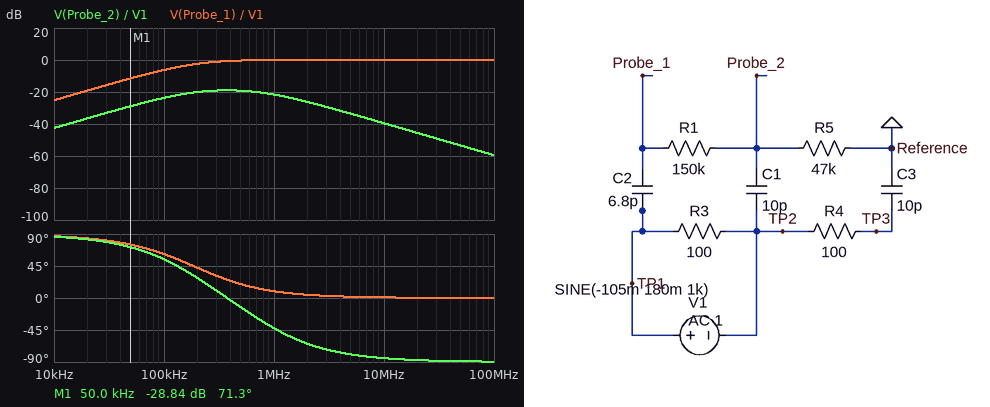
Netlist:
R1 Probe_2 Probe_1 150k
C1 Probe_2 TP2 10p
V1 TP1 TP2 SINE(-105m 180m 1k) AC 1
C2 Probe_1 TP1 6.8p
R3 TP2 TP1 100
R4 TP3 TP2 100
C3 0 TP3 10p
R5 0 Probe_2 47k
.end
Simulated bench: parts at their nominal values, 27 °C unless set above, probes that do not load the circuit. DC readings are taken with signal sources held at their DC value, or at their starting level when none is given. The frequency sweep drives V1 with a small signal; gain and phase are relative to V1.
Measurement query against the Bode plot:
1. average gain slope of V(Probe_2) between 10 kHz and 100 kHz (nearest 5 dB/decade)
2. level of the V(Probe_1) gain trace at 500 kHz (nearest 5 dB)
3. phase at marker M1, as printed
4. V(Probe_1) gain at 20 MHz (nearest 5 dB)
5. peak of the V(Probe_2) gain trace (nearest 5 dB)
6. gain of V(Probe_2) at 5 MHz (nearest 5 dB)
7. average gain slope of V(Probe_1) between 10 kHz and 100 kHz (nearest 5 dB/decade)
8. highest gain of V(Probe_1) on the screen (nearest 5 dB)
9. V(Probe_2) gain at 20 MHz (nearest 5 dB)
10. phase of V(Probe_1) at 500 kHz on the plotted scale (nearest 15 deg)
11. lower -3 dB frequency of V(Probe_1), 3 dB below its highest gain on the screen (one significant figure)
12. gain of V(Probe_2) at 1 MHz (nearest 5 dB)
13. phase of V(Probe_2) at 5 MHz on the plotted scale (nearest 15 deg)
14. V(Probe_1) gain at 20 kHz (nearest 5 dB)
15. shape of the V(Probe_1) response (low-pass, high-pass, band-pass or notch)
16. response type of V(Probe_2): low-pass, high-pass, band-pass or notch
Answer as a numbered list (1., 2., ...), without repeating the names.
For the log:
1. 20 dB/decade
2. 0 dB
3. 71.3 deg
4. 0 dB
5. -20 dB
6. -35 dB
7. 20 dB/decade
8. 0 dB
9. -45 dB
10. 15 deg
11. 200 kHz
12. -20 dB
13. -75 deg
14. -20 dB
15. high-pass
16. band-pass
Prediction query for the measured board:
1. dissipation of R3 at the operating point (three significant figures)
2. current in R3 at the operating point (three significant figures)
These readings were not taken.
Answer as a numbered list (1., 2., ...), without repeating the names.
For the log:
1. 110 µW
2. 1.05 mA
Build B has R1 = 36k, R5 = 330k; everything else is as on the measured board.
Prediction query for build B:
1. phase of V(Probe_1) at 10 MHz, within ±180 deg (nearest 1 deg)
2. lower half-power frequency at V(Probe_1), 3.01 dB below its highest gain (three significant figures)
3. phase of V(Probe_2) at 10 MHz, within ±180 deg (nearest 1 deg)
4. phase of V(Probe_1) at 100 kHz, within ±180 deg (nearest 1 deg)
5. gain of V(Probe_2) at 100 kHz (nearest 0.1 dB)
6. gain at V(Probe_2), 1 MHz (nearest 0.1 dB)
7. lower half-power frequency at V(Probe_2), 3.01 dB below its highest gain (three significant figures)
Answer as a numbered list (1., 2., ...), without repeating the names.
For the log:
1. 4 deg
2. 822 kHz
3. -83 deg
4. 42 deg
5. -10.0 dB
6. -10.6 dB
7. 66.9 kHz
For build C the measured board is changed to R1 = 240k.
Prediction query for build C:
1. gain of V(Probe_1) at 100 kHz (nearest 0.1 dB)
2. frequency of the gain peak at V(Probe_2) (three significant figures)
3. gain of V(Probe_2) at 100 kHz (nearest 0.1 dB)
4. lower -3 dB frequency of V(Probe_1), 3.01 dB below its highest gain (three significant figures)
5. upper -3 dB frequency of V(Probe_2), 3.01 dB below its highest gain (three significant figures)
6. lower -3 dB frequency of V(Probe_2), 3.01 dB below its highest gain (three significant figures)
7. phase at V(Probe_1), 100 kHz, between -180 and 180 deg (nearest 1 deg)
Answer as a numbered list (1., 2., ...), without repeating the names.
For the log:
1. -3.7 dB
2. 297 kHz
3. -24.8 dB
4. 116 kHz
5. 934 kHz
6. 94.5 kHz
7. 51 deg
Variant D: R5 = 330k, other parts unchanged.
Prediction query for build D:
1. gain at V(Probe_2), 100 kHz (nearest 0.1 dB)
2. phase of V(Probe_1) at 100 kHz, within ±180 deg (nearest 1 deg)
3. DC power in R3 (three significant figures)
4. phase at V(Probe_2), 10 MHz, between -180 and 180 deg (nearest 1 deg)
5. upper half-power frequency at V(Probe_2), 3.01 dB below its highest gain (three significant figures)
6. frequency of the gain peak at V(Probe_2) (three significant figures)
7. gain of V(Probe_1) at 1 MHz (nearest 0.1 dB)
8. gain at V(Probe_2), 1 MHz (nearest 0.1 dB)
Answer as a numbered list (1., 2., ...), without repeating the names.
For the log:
1. -10.9 dB
2. 42 deg
3. 110 µW
4. -88 deg
5. 408 kHz
6. 142 kHz
7. -0.2 dB
8. -19.9 dB
